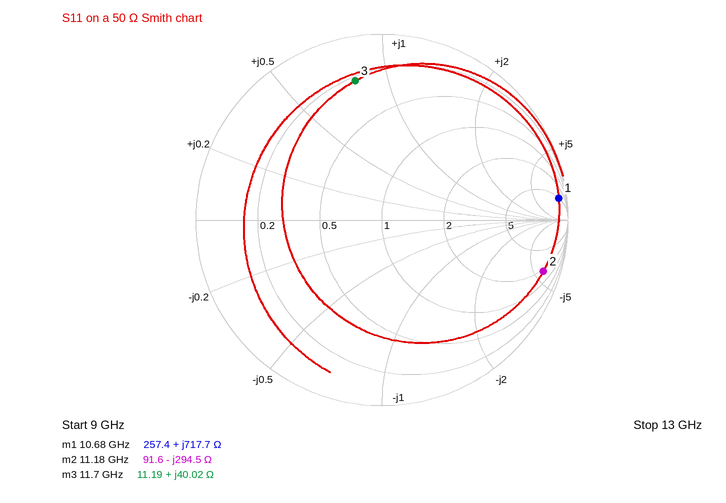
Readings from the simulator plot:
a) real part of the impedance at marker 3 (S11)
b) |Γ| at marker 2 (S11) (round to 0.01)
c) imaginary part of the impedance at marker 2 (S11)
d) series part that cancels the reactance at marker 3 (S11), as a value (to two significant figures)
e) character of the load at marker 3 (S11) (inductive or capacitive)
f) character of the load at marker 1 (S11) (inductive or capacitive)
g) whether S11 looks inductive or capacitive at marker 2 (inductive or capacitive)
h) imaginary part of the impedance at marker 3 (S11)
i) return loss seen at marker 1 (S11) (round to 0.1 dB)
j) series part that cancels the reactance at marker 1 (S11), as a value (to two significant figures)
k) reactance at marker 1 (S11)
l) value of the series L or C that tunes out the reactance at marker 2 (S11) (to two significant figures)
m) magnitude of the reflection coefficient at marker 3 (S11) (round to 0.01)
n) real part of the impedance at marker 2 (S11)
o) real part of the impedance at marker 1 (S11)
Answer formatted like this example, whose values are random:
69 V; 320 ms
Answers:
11.19 Ω; 0.91; -294.5 Ω; 340 fF; inductive; inductive; capacitive; +40.02 Ω; 0.4 dB; 21 fF; +717.7 Ω; 4.2 nH; 0.76; 91.6 Ω; 257.4 Ω
